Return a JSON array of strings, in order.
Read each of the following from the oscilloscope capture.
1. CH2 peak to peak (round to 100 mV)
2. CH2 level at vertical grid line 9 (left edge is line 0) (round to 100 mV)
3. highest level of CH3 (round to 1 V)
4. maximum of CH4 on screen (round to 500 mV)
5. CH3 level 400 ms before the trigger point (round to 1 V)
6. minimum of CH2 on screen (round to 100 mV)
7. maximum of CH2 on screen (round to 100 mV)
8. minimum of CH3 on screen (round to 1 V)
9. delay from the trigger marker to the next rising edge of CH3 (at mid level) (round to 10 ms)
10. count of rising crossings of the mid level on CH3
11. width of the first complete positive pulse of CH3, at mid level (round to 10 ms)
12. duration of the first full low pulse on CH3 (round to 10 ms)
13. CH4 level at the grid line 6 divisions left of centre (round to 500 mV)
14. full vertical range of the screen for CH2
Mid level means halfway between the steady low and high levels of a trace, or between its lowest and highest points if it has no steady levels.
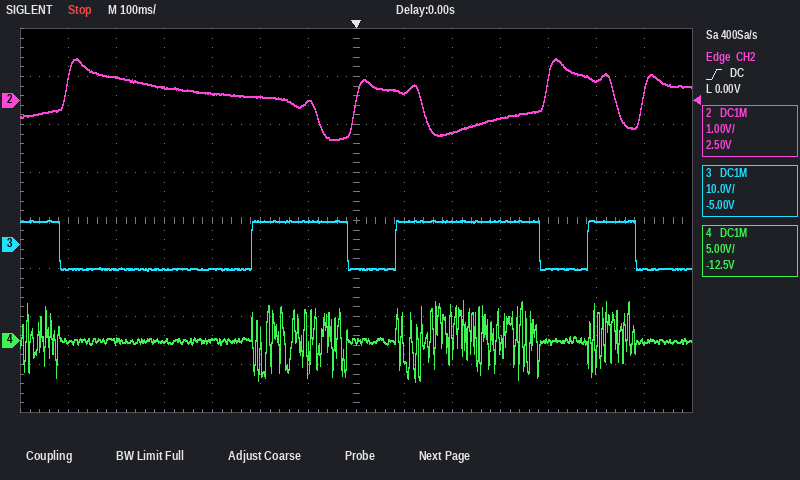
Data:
["1.7 V", "-700 mV", "5 V", "4.0 V", "-5 V", "-800 mV", "900 mV", "-5 V", "80 ms", "3", "200 ms", "400 ms", "0.0 V", "8 V"]
